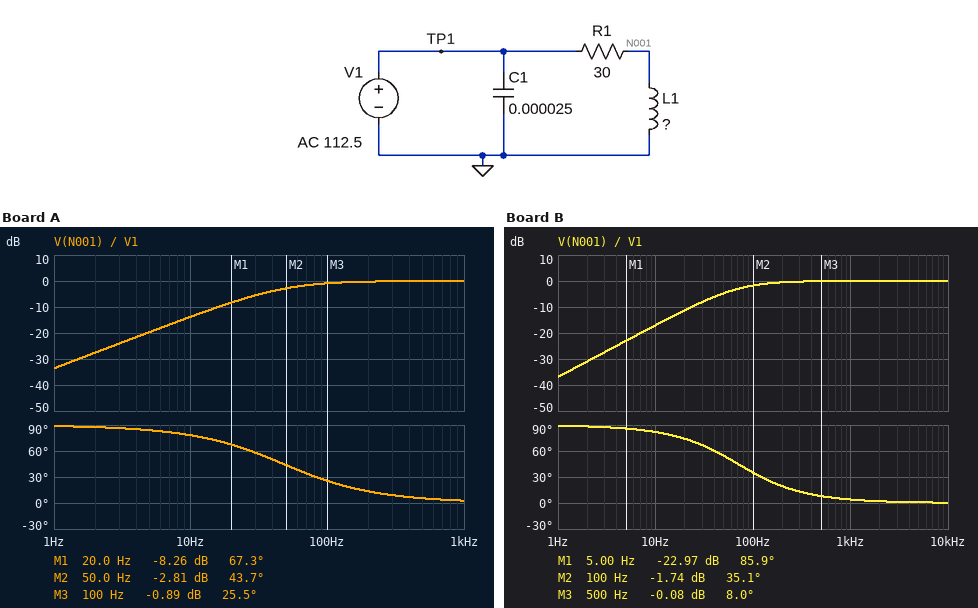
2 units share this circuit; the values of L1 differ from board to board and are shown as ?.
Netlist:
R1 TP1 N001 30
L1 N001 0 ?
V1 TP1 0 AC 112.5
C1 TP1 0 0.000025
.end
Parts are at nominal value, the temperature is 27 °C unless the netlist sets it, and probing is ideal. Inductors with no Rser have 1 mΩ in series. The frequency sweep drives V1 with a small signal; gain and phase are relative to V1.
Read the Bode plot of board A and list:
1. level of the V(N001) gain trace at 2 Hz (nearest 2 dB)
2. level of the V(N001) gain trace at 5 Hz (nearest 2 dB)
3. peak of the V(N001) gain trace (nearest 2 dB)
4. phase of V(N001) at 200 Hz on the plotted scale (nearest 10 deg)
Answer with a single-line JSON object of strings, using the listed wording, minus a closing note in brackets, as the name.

{"level of the V(N001) gain trace at 2 Hz": "-28 dB", "level of the V(N001) gain trace at 5 Hz": "-20 dB", "peak of the V(N001) gain trace": "0 dB", "phase of V(N001) at 200 Hz on the plotted scale": "10 deg"}
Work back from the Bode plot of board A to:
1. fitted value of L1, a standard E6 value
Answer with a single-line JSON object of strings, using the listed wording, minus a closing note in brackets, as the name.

{"fitted value of L1, a standard E6 value": "100 mH"}
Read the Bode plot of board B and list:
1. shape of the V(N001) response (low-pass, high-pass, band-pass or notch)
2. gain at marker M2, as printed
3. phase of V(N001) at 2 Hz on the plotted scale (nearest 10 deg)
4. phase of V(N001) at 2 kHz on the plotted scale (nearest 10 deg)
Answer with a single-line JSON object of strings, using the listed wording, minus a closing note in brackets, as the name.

{"shape of the V(N001) response": "high-pass", "gain at marker M2, as printed": "-1.74 dB", "phase of V(N001) at 2 Hz on the plotted scale": "90 deg", "phase of V(N001) at 2 kHz on the plotted scale": "0 deg"}
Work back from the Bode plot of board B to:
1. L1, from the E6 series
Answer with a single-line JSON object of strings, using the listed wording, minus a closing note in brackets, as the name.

{"L1, from the E6 series": "68 mH"}
